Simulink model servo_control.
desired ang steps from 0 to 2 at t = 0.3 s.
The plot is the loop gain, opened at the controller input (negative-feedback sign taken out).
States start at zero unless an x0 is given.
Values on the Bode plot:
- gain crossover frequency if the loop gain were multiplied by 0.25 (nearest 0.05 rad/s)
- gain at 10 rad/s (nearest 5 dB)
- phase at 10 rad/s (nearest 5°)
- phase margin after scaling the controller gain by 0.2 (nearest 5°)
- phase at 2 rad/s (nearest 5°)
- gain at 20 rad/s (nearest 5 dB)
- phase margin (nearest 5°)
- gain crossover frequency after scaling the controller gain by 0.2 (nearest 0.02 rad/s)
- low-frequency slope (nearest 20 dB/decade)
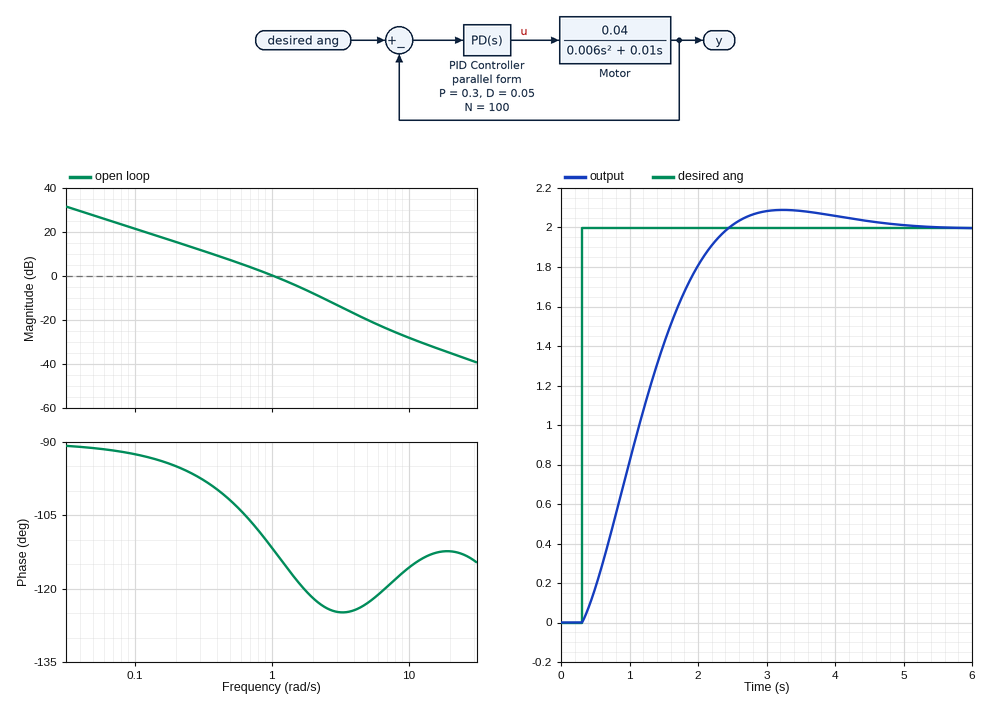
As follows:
0.30 rad/s
-30 dB
-115°
85°
-120°
-35 dB
70°
0.24 rad/s
-20 dB/decade
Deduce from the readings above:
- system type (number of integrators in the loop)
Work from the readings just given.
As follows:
1
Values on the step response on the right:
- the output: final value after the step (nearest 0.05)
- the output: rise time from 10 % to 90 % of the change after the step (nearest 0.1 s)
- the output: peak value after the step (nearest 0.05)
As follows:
2.00
1.5 s
2.10
